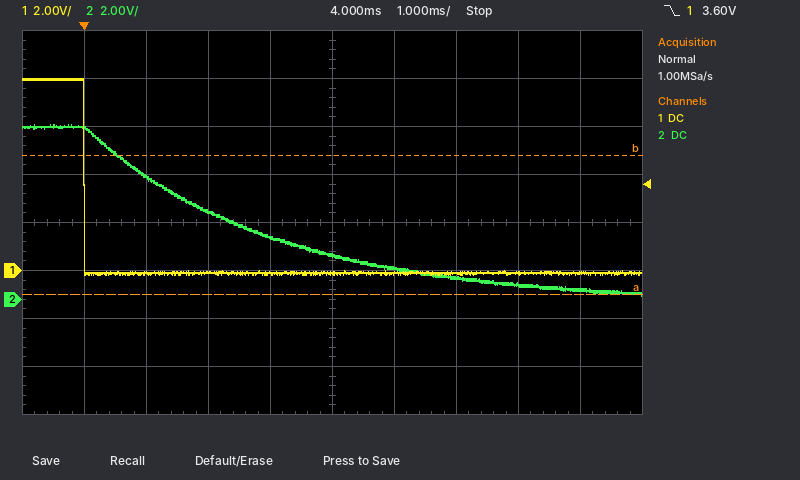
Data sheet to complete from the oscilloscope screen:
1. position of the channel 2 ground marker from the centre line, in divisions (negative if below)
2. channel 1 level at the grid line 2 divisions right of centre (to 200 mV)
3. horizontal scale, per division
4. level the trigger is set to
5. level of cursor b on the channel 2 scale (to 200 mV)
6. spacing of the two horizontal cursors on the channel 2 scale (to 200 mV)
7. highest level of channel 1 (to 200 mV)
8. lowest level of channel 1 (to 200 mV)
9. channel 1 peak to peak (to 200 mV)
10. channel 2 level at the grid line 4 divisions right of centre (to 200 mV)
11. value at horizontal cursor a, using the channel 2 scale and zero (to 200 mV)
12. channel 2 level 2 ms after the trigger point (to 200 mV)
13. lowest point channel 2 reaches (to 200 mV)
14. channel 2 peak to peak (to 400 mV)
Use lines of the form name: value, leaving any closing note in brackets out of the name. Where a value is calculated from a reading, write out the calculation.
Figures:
position of the channel 2 ground marker from the centre line, in divisions: -1.6 div
channel 1 level at the grid line 2 divisions right of centre: -200 mV
horizontal scale, per division: 1 ms
level the trigger is set to: 3.60 V
level of cursor b on the channel 2 scale: 6.0 V
spacing of the two horizontal cursors on the channel 2 scale: 5.8 V
highest level of channel 1: 8.0 V
lowest level of channel 1: -200 mV
channel 1 peak to peak: 8.0 V − (-200 mV) = 8.2 V
channel 2 level at the grid line 4 divisions right of centre: 400 mV
value at horizontal cursor a, using the channel 2 scale and zero: 200 mV
channel 2 level 2 ms after the trigger point: 3.6 V
lowest point channel 2 reaches: 200 mV
channel 2 peak to peak: 7.2 V
